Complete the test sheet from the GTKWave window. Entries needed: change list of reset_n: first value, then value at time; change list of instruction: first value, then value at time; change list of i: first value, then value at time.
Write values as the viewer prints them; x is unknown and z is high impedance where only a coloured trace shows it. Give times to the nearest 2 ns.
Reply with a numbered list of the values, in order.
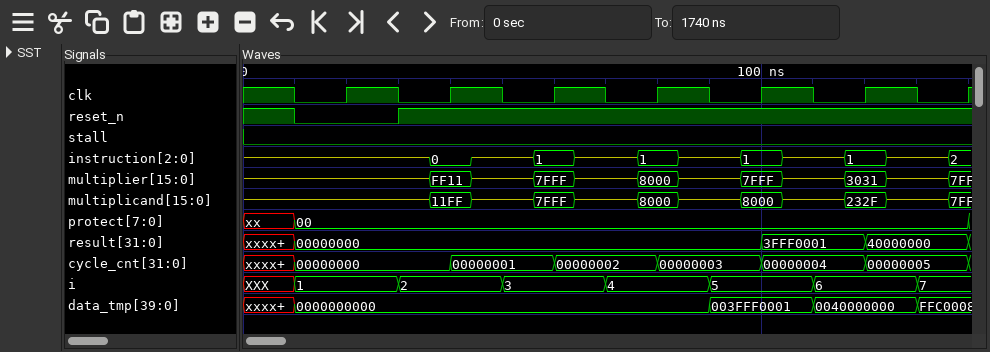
1. 1, 0 at 10 ns, 1 at 30 ns
2. z, 0 at 36 ns, z at 44 ns, 1 at 56 ns, z at 64 ns, 1 at 76 ns, z at 84 ns, 1 at 96 ns, z at 104 ns, 1 at 116 ns, z at 124 ns, 2 at 136 ns
3. XXX, 1 at 10 ns, 2 at 30 ns, 3 at 50 ns, 4 at 70 ns, 5 at 90 ns, 6 at 110 ns, 7 at 130 ns
